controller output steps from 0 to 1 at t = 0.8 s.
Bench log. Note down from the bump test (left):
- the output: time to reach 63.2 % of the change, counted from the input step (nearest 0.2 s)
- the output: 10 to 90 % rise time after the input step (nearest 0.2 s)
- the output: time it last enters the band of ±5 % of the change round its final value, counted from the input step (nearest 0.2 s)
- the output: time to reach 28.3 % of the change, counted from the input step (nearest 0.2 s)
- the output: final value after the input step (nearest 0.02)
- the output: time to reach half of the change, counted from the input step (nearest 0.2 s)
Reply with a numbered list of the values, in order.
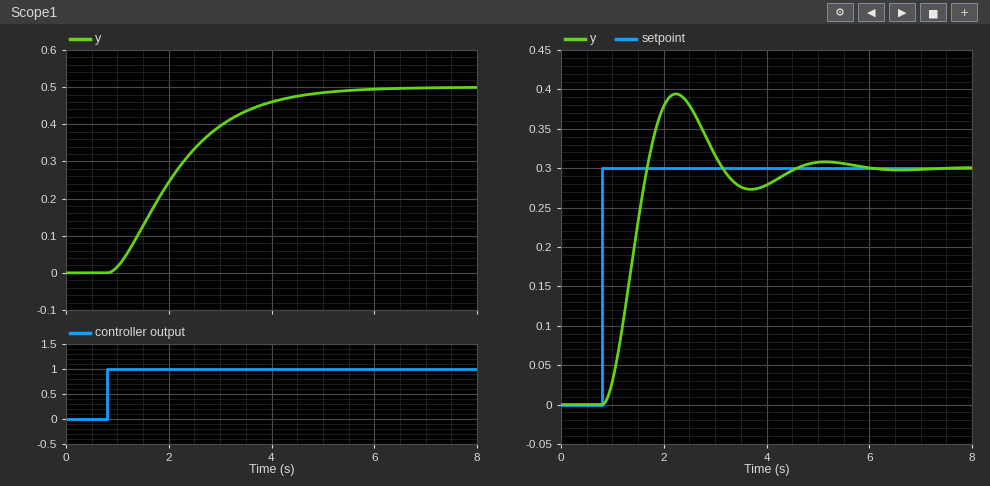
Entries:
1. 1.6 s
2. 2.6 s
3. 3.6 s
4. 0.8 s
5. 0.50
6. 1.2 s
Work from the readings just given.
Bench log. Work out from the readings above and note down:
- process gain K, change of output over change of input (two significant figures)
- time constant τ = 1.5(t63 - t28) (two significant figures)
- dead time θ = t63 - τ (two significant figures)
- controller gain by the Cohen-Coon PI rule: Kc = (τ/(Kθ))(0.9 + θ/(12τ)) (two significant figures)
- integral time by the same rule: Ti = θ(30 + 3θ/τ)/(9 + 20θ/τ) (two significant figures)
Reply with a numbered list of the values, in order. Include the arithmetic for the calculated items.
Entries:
1. (0.5 - 0) / 1 = 0.50
2. 1.5 × (1.6 - 0.8) = 1.2 s
3. 1.6 - 1.2 = 0.40 s
4. 1.2 / (0.5 × 0.4) × (0.9 + 0.4 / (12 × 1.2)) = 5.6
5. 0.4 × (30 + 3 × 0.4 / 1.2) / (9 + 20 × 0.4 / 1.2) = 0.79 s
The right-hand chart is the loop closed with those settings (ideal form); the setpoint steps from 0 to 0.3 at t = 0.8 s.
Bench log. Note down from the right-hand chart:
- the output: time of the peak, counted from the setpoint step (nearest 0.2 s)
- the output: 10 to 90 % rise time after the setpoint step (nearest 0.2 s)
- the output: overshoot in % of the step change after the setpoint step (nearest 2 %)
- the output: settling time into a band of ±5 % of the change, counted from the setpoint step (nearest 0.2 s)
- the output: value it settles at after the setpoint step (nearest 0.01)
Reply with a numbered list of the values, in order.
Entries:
1. 1.4 s
2. 0.6 s
3. 32 %
4. 3.4 s
5. 0.30
